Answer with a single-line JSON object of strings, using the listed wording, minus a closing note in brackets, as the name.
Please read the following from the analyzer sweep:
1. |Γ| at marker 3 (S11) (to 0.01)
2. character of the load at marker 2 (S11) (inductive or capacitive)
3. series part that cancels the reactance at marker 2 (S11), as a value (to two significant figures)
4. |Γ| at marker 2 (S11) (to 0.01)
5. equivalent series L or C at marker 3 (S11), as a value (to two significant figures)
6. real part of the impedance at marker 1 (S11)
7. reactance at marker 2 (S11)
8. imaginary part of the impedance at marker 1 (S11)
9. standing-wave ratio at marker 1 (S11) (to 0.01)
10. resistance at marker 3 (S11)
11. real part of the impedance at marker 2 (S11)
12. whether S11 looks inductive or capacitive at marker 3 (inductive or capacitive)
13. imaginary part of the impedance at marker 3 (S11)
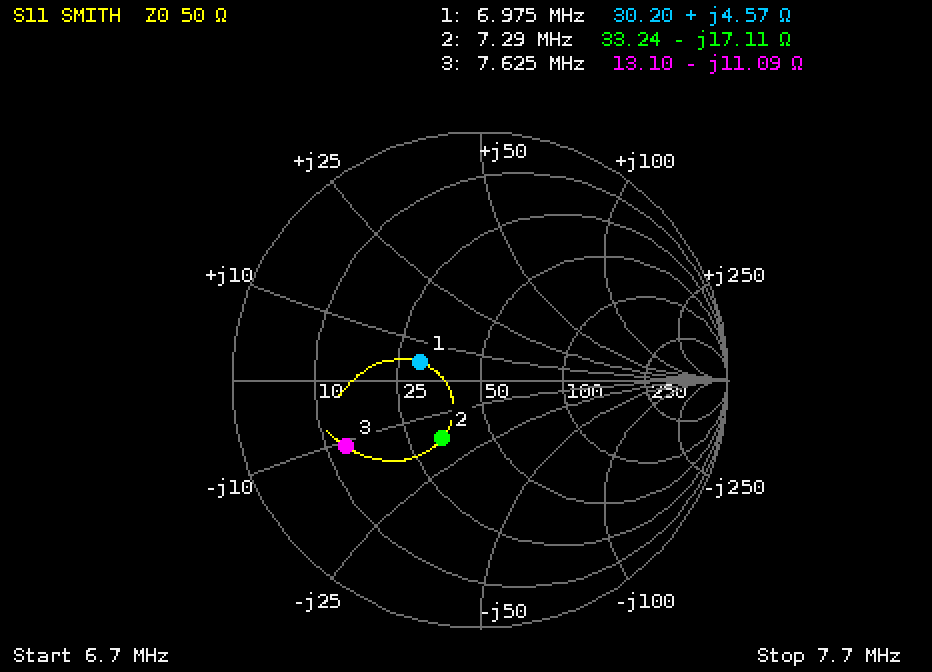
{"|Γ| at marker 3 (S11)": "0.60", "character of the load at marker 2 (S11)": "capacitive", "series part that cancels the reactance at marker 2 (S11), as a value": "370 nH", "|Γ| at marker 2 (S11)": "0.28", "equivalent series L or C at marker 3 (S11), as a value": "1.9 nF", "real part of the impedance at marker 1": "30.20 Ω", "reactance at marker 2": "-17.11 Ω", "imaginary part of the impedance at marker 1": "+4.57 Ω", "standing-wave ratio at marker 1 (S11)": "1.68", "resistance at marker 3": "13.10 Ω", "real part of the impedance at marker 2": "33.24 Ω", "whether S11 looks inductive or capacitive at marker 3": "capacitive", "imaginary part of the impedance at marker 3": "-11.09 Ω"}
